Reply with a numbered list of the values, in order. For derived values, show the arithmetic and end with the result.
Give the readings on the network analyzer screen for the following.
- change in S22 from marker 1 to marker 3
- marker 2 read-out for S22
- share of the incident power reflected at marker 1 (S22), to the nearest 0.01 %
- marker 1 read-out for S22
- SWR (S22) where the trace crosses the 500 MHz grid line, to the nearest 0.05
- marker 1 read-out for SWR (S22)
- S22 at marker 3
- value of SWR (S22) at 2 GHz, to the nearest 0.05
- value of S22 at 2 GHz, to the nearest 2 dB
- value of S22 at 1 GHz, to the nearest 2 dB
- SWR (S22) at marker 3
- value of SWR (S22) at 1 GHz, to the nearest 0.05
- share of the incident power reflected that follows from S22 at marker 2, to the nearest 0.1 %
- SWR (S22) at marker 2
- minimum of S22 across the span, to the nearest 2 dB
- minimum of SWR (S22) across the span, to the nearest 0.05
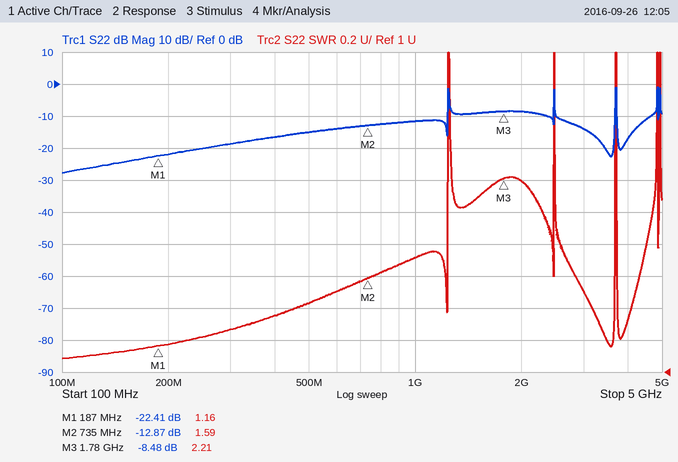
1. -8.48 − (-22.41) = 13.93 dB
2. -12.87 dB
3. 10^(-22.41/10) ≈ 0.57 %
4. -22.41 dB
5. 1.45
6. 1.16
7. -8.48 dB
8. 2.20
9. -8 dB
10. -12 dB
11. 2.21
12. 1.70
13. 10^(-12.87/10) ≈ 5.2 %
14. 1.59
15. -28 dB
16. 1.10
